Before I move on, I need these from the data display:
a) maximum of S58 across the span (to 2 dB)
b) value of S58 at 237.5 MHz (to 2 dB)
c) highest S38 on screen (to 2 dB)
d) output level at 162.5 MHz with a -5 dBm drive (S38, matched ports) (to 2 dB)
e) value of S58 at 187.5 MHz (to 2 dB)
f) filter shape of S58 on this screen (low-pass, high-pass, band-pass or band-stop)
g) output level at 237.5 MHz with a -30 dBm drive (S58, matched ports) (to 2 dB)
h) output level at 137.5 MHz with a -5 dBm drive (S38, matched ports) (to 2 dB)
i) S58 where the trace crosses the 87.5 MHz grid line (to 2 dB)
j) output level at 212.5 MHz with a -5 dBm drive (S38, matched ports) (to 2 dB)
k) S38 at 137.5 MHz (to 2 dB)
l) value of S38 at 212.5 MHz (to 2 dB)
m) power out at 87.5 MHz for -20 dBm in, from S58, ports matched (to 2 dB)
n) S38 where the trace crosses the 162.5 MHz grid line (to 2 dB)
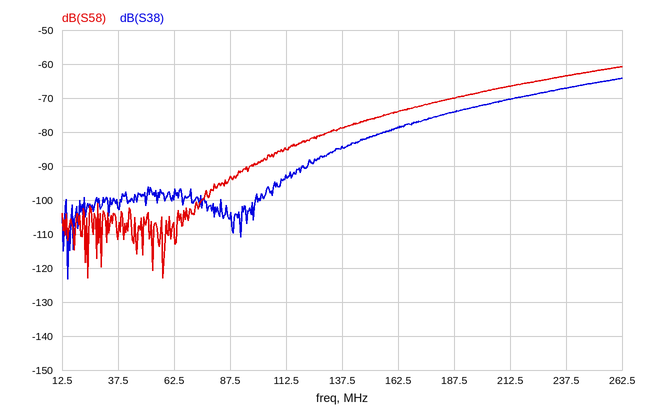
-60 dB
-64 dB
-64 dB
-84 dBm
-70 dB
high-pass
-94 dBm
-90 dBm
-94 dB
-76 dBm
-84 dB
-70 dB
-114 dBm
-78 dB
